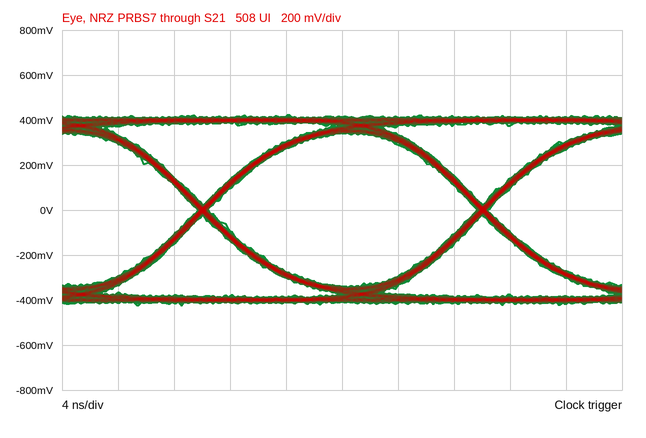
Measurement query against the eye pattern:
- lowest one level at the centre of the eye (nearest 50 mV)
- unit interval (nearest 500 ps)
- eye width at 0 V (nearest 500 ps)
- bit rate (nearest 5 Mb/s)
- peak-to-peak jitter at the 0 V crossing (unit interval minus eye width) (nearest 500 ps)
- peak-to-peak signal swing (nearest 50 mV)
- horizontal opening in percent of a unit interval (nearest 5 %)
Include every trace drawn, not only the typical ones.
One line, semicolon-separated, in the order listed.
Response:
350 mV; 20.0 ns; 19.0 ns; 50 Mb/s; 1.0 ns; 850 mV; 95 %
